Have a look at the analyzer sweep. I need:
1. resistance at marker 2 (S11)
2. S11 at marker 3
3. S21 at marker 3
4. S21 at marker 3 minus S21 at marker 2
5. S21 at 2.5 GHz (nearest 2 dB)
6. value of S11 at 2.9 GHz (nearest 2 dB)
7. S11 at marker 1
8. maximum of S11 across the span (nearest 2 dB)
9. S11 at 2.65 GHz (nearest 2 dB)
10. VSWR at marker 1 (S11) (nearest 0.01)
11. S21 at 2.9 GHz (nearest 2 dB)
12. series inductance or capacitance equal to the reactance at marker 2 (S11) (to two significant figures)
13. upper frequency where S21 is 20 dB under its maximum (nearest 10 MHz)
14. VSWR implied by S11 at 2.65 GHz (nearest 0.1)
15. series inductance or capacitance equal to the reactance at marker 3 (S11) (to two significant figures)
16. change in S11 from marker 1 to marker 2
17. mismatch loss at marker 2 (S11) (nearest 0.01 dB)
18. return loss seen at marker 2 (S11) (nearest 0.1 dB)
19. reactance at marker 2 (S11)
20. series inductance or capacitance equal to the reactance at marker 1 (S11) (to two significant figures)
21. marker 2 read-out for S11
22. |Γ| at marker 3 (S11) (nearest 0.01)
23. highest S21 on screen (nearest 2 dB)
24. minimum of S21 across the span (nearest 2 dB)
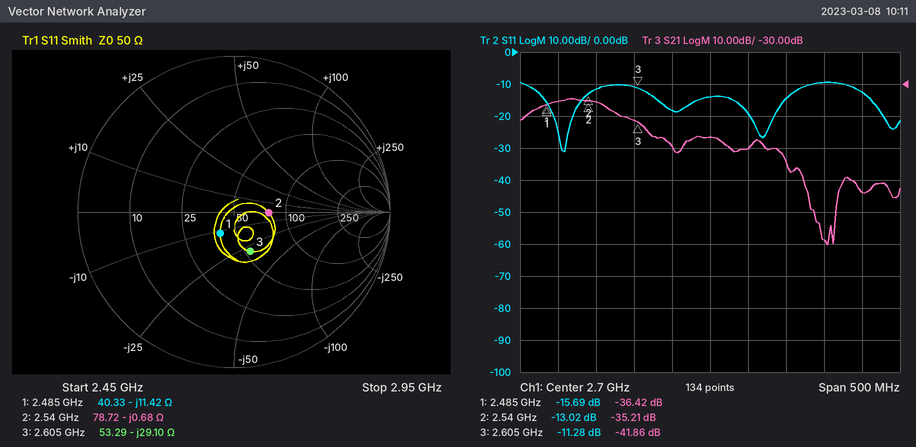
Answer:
78.72 Ω
-11.28 dB
-41.86 dB
-6.65 dB
-36 dB
-12 dB
-15.69 dB
-10 dB
-18 dB
1.39
-64 dB
92 pF
2.80 GHz
1.3
2.1 pF
2.67 dB
0.22 dB
13.0 dB
-0.68 Ω
5.6 pF
-13.02 dB
0.27
-34 dB
-80 dB
